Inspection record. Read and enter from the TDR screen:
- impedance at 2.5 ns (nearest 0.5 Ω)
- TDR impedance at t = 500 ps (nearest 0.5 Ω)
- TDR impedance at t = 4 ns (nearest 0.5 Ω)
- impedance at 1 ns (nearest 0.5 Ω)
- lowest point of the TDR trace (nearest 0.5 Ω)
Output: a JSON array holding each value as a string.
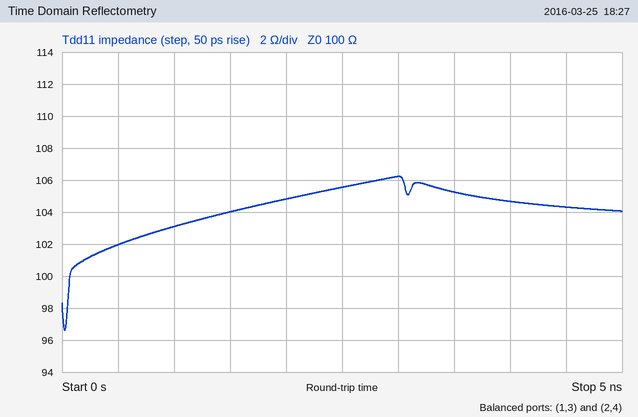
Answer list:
["105.5 Ω", "102.0 Ω", "104.5 Ω", "103.0 Ω", "96.5 Ω"]
